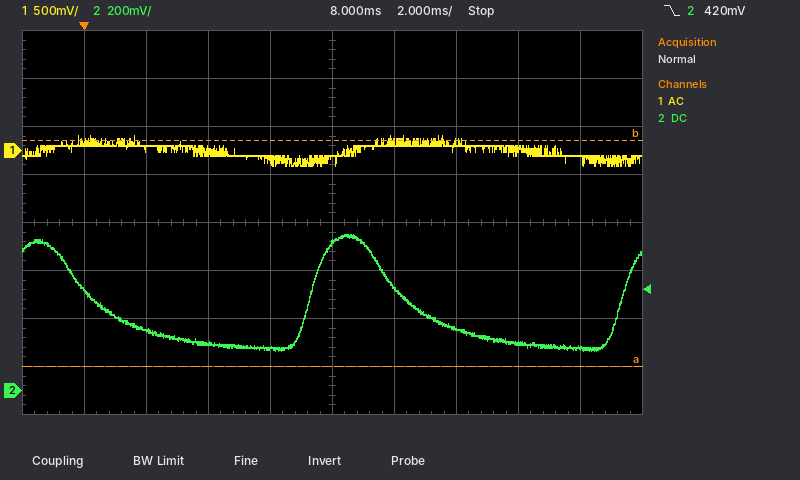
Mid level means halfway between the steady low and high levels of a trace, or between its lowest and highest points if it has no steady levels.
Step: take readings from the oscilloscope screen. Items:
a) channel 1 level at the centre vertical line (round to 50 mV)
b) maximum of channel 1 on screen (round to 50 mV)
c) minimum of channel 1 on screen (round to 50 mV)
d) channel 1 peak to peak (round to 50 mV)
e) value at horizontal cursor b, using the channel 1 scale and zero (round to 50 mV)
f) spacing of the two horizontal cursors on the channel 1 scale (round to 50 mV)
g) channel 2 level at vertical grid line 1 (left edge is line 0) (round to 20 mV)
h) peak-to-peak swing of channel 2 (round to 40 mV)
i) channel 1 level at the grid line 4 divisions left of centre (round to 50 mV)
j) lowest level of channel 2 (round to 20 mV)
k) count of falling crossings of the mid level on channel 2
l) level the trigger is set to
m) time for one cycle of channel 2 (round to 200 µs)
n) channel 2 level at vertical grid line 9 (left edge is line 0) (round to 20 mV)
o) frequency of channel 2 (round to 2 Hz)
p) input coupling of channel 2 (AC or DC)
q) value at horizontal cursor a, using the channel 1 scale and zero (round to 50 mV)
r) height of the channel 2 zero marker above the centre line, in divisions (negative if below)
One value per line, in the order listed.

-50 mV
150 mV
-150 mV
300 mV
100 mV
2.35 V
420 mV
480 mV
100 mV
160 mV
2
420 mV
10.0 ms
180 mV
100 Hz
DC
-2.25 V
-3.5 div
